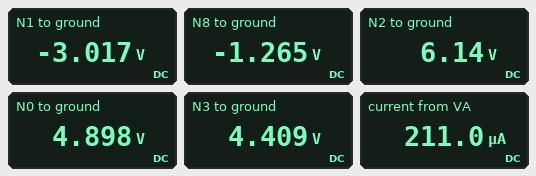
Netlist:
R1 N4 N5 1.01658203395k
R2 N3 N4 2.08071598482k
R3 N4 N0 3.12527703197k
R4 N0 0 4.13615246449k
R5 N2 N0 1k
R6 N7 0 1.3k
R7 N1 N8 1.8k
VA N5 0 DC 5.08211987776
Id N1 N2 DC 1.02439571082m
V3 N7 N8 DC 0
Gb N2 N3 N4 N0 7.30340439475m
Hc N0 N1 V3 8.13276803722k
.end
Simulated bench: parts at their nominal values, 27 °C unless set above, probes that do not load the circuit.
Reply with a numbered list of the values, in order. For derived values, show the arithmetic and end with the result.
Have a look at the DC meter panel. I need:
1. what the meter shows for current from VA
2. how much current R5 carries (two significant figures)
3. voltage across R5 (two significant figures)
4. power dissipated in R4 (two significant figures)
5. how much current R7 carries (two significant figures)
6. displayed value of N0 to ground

1. 211.0 µA
2. (6.14 V - 4.898 V) / 1 kΩ = 1.2 mA
3. 6.14 V - 4.898 V = 1.2 V
4. (4.898 V)^2 / 4.136 kΩ = 5.8 mW
5. (-1.265 V - (-3.017 V)) / 1.8 kΩ = 970 µA
6. 4.898 V
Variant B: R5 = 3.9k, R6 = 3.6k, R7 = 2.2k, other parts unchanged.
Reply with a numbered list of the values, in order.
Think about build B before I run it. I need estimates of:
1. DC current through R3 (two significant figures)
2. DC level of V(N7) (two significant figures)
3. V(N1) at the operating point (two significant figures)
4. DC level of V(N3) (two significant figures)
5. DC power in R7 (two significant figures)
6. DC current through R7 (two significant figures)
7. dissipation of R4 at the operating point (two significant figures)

1. 52 µA
2. -9.4 V
3. -15 V
4. 8.7 V
5. 15 mW
6. 2.6 mA
7. 8.9 mW
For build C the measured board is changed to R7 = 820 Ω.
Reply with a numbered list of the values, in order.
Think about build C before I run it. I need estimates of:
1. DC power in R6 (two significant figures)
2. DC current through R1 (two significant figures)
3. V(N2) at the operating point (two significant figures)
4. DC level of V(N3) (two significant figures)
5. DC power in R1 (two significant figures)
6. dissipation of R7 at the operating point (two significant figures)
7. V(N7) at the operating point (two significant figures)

1. 820 µW
2. 360 µA
3. 6.2 V
4. 3.9 V
5. 130 µW
6. 520 µW
7. -1.0 V
